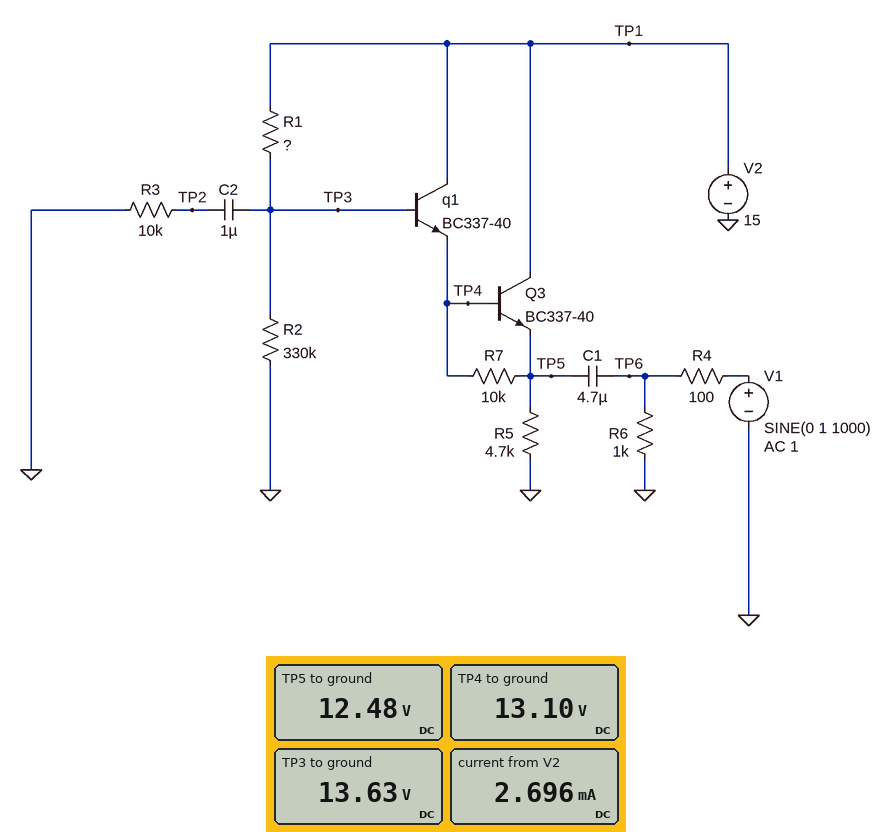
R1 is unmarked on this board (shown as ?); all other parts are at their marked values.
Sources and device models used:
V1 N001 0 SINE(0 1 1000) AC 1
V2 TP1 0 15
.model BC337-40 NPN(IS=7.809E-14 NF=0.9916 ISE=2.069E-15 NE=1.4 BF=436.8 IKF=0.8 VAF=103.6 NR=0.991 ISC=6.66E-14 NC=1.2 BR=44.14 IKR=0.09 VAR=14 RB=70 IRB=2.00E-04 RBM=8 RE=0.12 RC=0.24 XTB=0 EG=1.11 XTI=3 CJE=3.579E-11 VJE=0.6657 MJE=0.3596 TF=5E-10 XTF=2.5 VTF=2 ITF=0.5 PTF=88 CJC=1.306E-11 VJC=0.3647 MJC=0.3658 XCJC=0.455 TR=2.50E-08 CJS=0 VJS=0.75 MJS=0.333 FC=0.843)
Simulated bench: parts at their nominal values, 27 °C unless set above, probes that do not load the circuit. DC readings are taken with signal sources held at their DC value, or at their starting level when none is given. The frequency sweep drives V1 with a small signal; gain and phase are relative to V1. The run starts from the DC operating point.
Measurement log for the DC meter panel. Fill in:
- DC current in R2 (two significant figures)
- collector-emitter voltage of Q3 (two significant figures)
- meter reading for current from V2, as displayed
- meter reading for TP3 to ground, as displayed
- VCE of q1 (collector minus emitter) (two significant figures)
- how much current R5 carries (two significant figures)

41 µA
2.5 V
2.696 mA
13.63 V
1.9 V
2.7 mA
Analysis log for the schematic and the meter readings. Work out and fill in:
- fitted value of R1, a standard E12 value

33 kΩ
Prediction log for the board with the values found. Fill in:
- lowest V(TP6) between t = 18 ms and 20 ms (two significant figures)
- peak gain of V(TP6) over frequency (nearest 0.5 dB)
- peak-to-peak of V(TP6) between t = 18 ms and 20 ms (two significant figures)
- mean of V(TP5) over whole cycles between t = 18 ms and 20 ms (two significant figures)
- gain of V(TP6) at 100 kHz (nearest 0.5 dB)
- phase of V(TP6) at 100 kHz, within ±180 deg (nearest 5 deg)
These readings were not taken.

-470 mV
-1.0 dB
1.1 V
13 V
-20.0 dB
0 deg
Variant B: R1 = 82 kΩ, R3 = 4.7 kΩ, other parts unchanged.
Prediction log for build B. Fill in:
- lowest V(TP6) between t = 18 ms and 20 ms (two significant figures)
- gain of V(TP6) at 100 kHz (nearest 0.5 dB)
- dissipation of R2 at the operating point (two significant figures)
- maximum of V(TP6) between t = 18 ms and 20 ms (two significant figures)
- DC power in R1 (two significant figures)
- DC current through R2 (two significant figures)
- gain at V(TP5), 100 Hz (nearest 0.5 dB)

-490 mV
-19.0 dB
440 µW
680 mV
110 µW
36 µA
-29.5 dB
